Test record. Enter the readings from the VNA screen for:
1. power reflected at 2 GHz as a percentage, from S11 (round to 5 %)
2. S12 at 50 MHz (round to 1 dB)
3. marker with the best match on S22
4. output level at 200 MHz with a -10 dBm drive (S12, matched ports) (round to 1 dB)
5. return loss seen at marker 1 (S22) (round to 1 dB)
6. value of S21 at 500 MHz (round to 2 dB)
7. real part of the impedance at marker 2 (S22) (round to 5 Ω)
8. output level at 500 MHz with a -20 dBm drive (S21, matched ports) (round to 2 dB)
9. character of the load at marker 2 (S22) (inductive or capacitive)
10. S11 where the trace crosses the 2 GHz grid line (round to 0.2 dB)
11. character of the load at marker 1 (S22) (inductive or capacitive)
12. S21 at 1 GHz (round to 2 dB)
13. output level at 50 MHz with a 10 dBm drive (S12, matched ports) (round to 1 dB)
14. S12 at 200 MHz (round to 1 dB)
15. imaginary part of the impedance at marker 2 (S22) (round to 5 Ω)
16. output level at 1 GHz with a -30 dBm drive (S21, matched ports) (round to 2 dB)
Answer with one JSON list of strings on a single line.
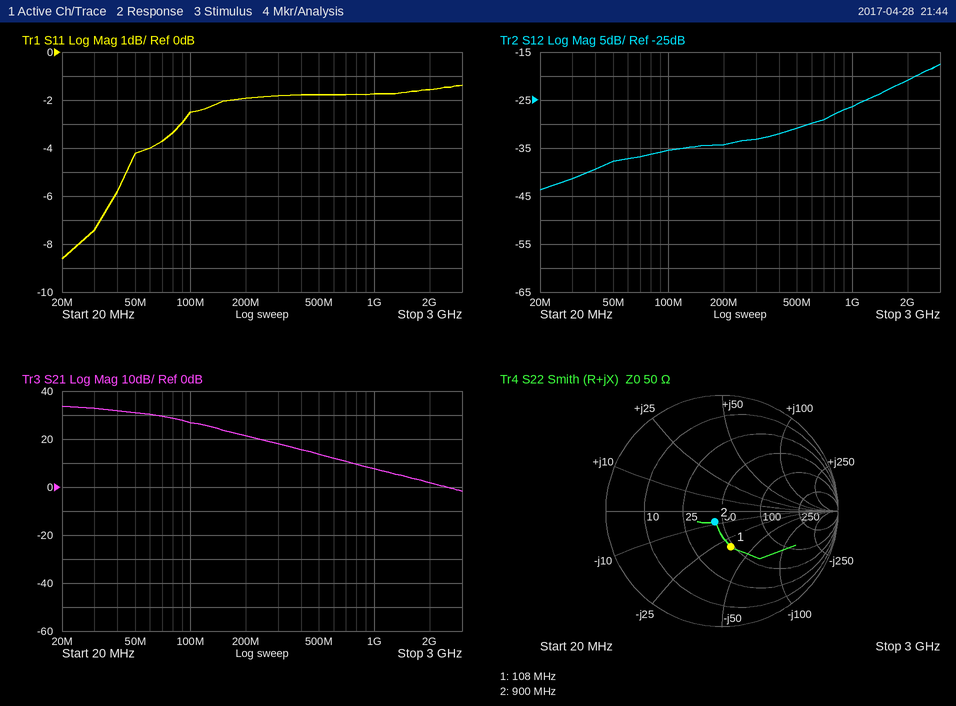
["70 %", "-38 dB", "marker 2", "-44 dBm", "10 dB", "14 dB", "45 Ω", "-6 dBm", "capacitive", "-1.6 dB", "capacitive", "8 dB", "-28 dBm", "-34 dB", "-10 Ω", "-22 dBm"]
